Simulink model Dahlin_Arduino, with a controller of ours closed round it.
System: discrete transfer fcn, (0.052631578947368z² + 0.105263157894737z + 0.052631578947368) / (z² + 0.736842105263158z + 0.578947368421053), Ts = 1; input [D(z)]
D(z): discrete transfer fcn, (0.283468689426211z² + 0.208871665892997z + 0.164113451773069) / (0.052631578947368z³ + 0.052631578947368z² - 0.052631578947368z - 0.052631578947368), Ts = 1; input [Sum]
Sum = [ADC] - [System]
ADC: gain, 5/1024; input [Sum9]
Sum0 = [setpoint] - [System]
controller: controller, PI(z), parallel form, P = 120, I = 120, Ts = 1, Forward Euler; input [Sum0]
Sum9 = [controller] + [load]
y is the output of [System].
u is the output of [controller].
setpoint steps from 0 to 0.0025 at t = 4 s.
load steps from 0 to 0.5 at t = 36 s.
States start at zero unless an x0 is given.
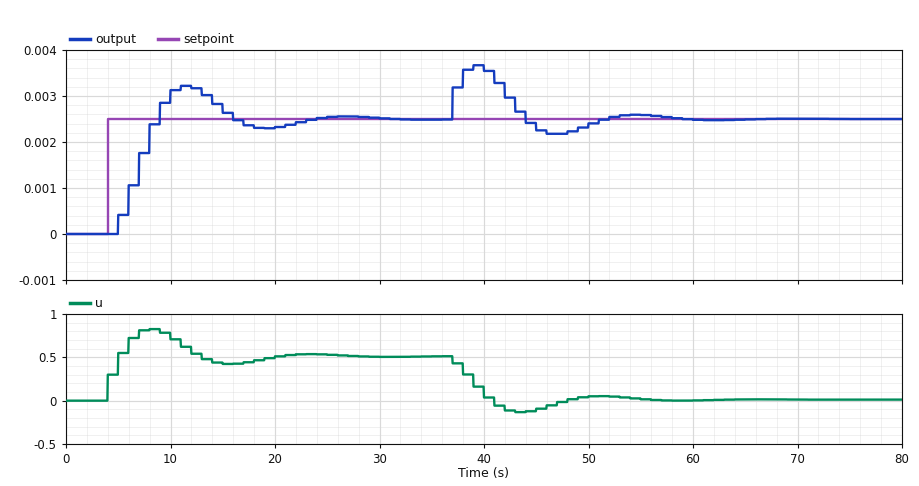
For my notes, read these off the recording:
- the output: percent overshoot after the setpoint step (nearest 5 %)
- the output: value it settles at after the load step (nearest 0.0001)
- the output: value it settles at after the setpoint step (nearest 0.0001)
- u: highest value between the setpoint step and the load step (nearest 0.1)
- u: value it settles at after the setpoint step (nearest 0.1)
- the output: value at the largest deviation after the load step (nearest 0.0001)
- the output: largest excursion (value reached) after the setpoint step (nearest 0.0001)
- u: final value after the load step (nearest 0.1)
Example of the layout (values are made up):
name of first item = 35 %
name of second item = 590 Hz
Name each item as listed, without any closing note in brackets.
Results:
the output: percent overshoot after the setpoint step = 30 %
the output: value it settles at after the load step = 0.0025
the output: value it settles at after the setpoint step = 0.0025
u: highest value between the setpoint step and the load step = 0.8
u: value it settles at after the setpoint step = 0.5
the output: value at the largest deviation after the load step = 0.0037
the output: largest excursion (value reached) after the setpoint step = 0.0032
u: final value after the load step = 0.0
